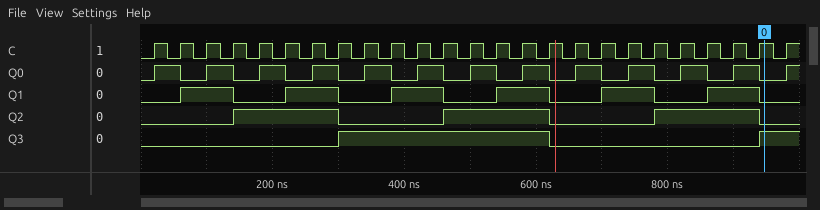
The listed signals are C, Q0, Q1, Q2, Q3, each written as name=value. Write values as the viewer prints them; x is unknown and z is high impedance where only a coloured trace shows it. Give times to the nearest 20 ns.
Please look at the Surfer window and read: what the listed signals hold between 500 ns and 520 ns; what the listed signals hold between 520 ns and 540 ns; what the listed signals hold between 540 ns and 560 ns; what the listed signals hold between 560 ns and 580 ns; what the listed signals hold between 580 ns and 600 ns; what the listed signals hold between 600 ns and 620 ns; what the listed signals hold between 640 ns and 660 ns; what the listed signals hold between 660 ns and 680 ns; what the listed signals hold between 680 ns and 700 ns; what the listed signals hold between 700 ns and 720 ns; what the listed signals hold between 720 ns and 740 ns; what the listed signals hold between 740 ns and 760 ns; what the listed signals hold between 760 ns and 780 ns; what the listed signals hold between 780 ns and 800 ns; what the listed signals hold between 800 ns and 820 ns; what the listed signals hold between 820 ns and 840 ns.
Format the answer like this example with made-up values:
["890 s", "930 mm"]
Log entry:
["C=1, Q0=1, Q1=0, Q2=1, Q3=1", "C=0, Q0=1, Q1=0, Q2=1, Q3=1", "C=1, Q0=0, Q1=1, Q2=1, Q3=1", "C=0, Q0=0, Q1=1, Q2=1, Q3=1", "C=1, Q0=1, Q1=1, Q2=1, Q3=1", "C=0, Q0=1, Q1=1, Q2=1, Q3=1", "C=0, Q0=0, Q1=0, Q2=0, Q3=0", "C=1, Q0=1, Q1=0, Q2=0, Q3=0", "C=0, Q0=1, Q1=0, Q2=0, Q3=0", "C=1, Q0=0, Q1=1, Q2=0, Q3=0", "C=0, Q0=0, Q1=1, Q2=0, Q3=0", "C=1, Q0=1, Q1=1, Q2=0, Q3=0", "C=0, Q0=1, Q1=1, Q2=0, Q3=0", "C=1, Q0=0, Q1=0, Q2=1, Q3=0", "C=0, Q0=0, Q1=0, Q2=1, Q3=0", "C=1, Q0=1, Q1=0, Q2=1, Q3=0"]
